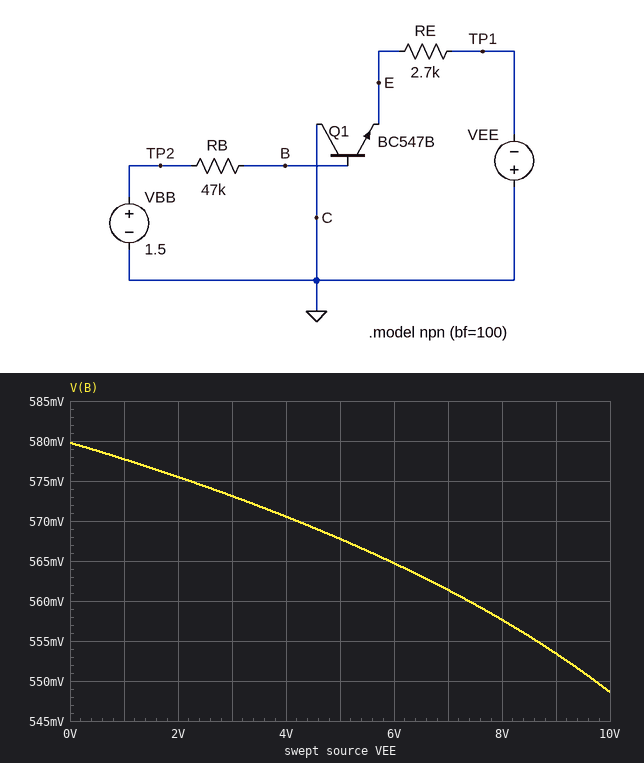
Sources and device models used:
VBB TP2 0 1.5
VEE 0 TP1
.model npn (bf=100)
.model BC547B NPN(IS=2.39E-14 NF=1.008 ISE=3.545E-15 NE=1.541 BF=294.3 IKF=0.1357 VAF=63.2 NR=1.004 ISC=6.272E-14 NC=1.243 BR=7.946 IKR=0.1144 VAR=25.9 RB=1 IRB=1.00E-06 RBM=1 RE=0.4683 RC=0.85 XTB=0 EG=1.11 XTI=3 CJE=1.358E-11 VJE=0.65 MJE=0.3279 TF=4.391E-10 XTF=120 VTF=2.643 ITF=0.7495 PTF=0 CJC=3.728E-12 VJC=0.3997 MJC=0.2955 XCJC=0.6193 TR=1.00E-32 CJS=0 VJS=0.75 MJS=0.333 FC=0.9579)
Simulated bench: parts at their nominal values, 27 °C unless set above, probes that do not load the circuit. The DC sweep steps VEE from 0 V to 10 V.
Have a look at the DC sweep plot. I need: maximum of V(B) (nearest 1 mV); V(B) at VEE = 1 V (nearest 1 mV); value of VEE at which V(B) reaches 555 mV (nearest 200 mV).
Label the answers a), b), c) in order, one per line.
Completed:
a) 580 mV
b) 578 mV
c) 8.6 V
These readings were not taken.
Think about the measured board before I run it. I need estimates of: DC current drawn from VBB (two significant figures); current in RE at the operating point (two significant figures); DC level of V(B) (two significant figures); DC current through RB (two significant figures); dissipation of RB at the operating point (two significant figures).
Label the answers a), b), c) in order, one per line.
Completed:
a) 20 µA
b) 750 nA
c) 580 mV
d) 20 µA
e) 18 µW
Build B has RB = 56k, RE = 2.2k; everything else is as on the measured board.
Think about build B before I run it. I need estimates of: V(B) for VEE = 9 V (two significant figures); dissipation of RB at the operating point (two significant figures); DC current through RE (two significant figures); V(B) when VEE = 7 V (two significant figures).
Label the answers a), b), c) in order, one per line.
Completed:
a) 520 mV
b) 15 µW
c) 880 nA
d) 540 mV
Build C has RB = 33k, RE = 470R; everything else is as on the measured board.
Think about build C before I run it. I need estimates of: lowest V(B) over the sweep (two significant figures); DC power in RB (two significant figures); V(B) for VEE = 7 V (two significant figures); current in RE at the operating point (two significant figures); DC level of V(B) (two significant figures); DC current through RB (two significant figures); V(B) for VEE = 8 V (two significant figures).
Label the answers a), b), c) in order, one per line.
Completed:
a) -820 mV
b) 25 µW
c) -150 mV
d) 3.5 µA
e) 590 mV
f) 28 µA
g) -370 mV
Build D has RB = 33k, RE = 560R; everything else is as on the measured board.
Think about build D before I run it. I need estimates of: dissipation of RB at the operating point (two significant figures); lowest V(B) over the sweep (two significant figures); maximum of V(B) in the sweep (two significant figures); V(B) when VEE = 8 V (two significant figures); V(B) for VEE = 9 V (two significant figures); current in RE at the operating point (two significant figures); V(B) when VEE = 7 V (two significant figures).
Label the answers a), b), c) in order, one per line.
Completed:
a) 25 µW
b) -500 mV
c) 590 mV
d) -120 mV
e) -310 mV
f) 3.1 µA
g) 75 mV
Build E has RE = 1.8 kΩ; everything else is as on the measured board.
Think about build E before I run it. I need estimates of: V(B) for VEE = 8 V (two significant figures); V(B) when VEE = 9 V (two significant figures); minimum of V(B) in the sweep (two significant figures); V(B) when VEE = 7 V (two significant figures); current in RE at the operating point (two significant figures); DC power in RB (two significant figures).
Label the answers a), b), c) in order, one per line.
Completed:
a) 540 mV
b) 520 mV
c) 500 mV
d) 550 mV
e) 1.1 µA
f) 18 µW
